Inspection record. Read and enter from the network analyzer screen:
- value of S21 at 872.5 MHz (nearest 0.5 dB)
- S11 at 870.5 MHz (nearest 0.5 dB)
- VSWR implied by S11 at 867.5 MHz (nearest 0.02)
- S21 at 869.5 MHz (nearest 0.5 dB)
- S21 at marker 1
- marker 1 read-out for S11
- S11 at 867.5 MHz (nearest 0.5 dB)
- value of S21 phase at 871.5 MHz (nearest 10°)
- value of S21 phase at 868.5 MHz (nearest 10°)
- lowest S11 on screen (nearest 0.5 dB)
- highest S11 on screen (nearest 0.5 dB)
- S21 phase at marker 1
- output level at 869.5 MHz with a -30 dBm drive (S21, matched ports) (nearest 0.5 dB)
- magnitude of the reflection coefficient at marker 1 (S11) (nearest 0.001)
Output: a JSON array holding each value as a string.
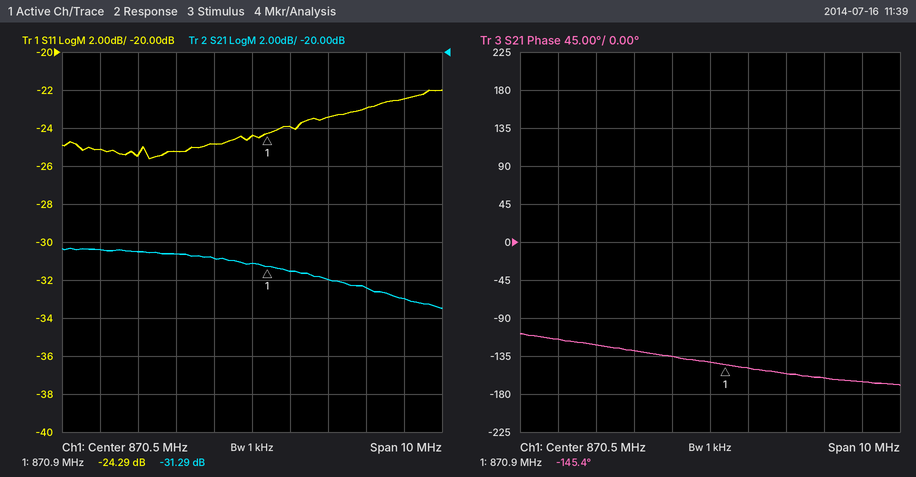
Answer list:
["-32.0 dB", "-24.5 dB", "1.12", "-31.0 dB", "-31.29 dB", "-24.29 dB", "-25.5 dB", "-150°", "-130°", "-25.5 dB", "-22.0 dB", "-145.4°", "-61.0 dBm", "0.061"]
